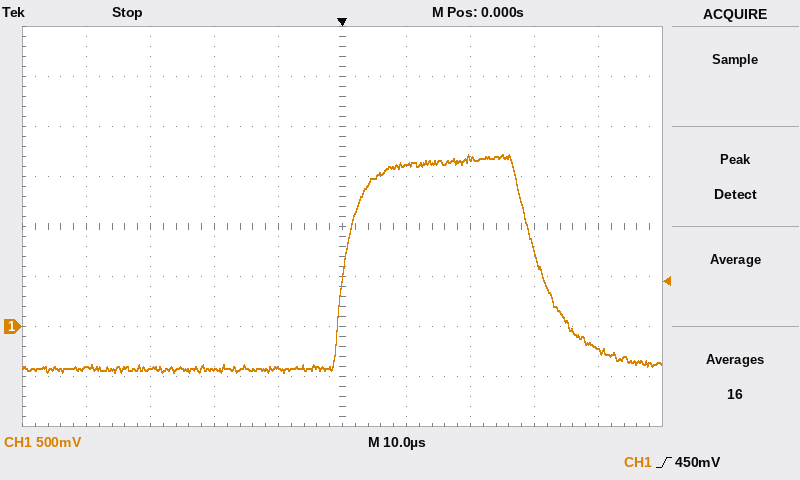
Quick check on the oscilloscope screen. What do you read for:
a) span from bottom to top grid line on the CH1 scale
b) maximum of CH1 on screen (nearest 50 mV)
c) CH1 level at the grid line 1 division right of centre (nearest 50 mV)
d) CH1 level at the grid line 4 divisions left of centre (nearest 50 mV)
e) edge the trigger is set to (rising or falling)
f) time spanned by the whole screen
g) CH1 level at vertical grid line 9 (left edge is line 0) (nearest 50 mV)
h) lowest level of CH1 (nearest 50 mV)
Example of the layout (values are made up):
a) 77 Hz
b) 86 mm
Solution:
a) 4 V
b) 1.70 V
c) 1.60 V
d) -400 mV
e) rising
f) 100 µs
g) -250 mV
h) -450 mV
